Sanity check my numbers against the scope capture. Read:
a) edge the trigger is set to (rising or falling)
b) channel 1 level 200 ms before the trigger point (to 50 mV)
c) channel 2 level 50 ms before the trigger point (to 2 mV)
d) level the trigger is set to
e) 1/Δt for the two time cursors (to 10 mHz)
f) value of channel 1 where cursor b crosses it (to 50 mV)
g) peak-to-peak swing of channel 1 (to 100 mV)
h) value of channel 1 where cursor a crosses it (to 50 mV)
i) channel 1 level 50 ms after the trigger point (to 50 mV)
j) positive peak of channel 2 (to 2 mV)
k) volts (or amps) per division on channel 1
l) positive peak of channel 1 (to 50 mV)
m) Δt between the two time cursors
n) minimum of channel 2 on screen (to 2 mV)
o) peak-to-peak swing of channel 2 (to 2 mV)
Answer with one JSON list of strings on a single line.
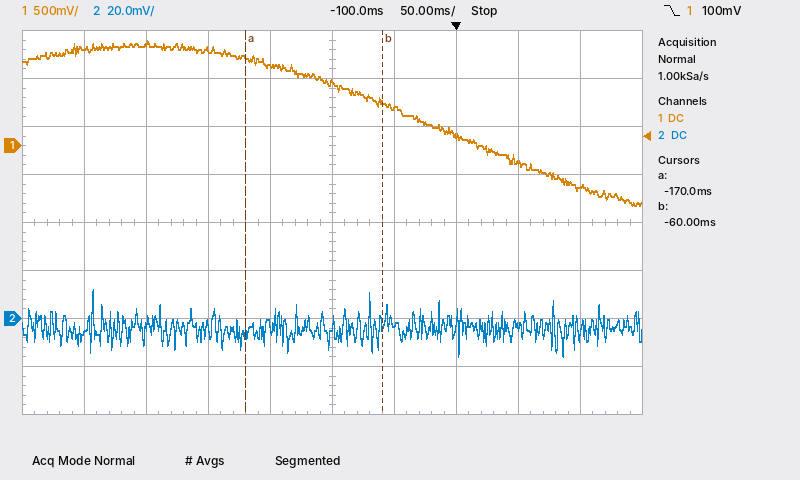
["falling", "1.00 V", "-2 mV", "100 mV", "9.09 Hz", "450 mV", "1.70 V", "900 mV", "-200 mV", "12 mV", "500 mV", "1.10 V", "110 ms", "-16 mV", "28 mV"]
